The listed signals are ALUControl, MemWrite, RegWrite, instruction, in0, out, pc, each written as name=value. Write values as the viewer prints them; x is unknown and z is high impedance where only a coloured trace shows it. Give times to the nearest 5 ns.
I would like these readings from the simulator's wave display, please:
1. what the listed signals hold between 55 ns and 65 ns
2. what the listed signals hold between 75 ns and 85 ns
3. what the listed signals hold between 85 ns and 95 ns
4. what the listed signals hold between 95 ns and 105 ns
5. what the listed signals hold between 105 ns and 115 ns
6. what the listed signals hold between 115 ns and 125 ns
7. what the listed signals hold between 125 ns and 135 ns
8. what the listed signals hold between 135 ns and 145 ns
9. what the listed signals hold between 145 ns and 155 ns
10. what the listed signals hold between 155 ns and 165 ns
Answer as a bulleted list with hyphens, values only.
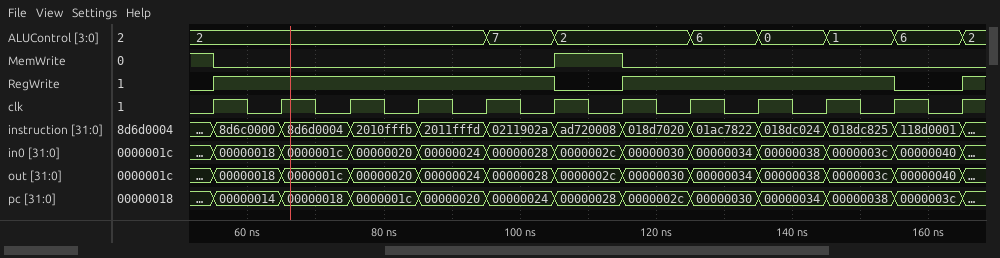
- ALUControl=2, MemWrite=0, RegWrite=1, instruction=8d6c0000, in0=00000018, out=00000018, pc=00000014
- ALUControl=2, MemWrite=0, RegWrite=1, instruction=2010fffb, in0=00000020, out=00000020, pc=0000001c
- ALUControl=2, MemWrite=0, RegWrite=1, instruction=2011fffd, in0=00000024, out=00000024, pc=00000020
- ALUControl=7, MemWrite=0, RegWrite=1, instruction=0211902a, in0=00000028, out=00000028, pc=00000024
- ALUControl=2, MemWrite=1, RegWrite=0, instruction=ad720008, in0=0000002c, out=0000002c, pc=00000028
- ALUControl=2, MemWrite=0, RegWrite=1, instruction=018d7020, in0=00000030, out=00000030, pc=0000002c
- ALUControl=6, MemWrite=0, RegWrite=1, instruction=01ac7822, in0=00000034, out=00000034, pc=00000030
- ALUControl=0, MemWrite=0, RegWrite=1, instruction=018dc024, in0=00000038, out=00000038, pc=00000034
- ALUControl=1, MemWrite=0, RegWrite=1, instruction=018dc825, in0=0000003c, out=0000003c, pc=00000038
- ALUControl=6, MemWrite=0, RegWrite=0, instruction=118d0001, in0=00000040, out=00000040, pc=0000003c
